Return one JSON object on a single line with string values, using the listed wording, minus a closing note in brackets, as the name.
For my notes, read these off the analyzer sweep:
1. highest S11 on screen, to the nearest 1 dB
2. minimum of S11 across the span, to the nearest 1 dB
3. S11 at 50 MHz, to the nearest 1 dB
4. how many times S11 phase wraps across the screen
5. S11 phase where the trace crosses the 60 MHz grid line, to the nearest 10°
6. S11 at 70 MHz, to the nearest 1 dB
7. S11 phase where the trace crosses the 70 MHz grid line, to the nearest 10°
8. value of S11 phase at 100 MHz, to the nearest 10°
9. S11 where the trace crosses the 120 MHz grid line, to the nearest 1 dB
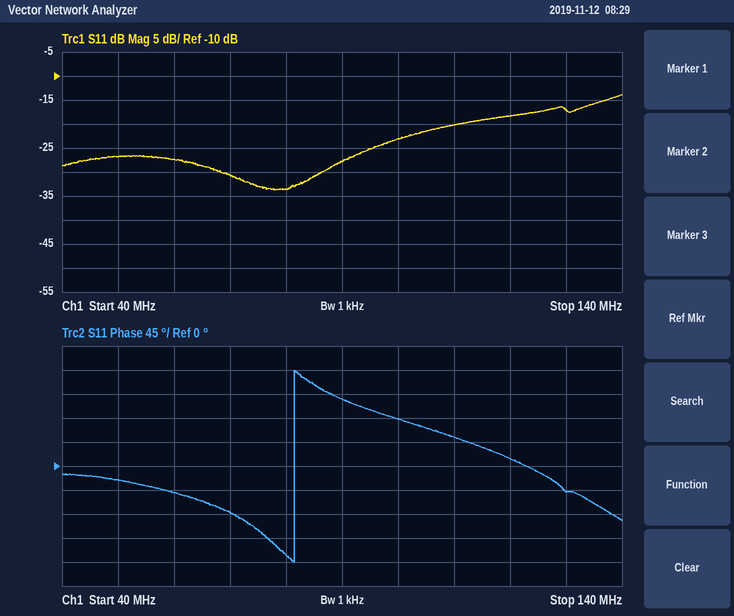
{"highest S11 on screen, to the nearest 1 dB": "-14 dB", "minimum of S11 across the span, to the nearest 1 dB": "-34 dB", "S11 at 50 MHz, to the nearest 1 dB": "-27 dB", "how many times S11 phase wraps across the screen": "1", "S11 phase where the trace crosses the 60 MHz grid line, to the nearest 10°": "-50°", "S11 at 70 MHz, to the nearest 1 dB": "-31 dB", "S11 phase where the trace crosses the 70 MHz grid line, to the nearest 10°": "-90°", "value of S11 phase at 100 MHz, to the nearest 10°": "90°", "S11 where the trace crosses the 120 MHz grid line, to the nearest 1 dB": "-18 dB"}
